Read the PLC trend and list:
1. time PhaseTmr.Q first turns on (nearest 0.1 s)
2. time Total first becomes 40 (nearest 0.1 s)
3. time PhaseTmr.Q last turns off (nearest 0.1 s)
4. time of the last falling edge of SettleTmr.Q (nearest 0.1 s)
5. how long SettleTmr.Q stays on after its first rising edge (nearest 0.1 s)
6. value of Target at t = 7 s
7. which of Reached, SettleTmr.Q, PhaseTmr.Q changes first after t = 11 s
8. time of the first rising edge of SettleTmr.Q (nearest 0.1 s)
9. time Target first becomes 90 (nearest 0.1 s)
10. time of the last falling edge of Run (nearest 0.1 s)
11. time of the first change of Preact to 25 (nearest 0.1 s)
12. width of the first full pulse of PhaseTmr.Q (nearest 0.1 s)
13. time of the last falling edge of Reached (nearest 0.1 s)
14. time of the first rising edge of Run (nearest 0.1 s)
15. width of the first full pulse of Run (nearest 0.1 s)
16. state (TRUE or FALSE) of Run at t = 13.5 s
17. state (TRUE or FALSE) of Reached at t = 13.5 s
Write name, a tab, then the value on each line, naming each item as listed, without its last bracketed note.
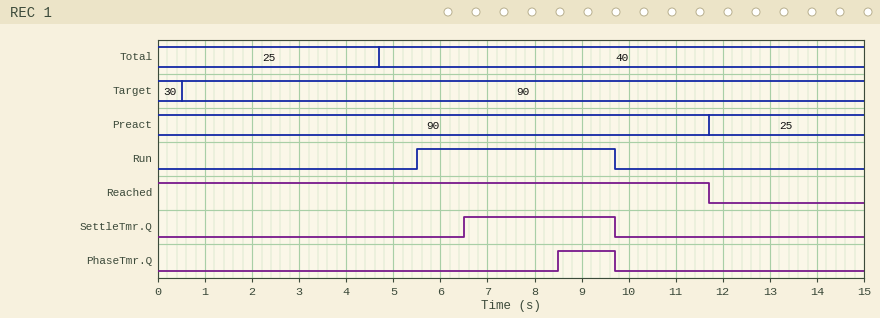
time PhaseTmr.Q first turns on	8.5 s
time Total first becomes 40	4.7 s
time PhaseTmr.Q last turns off	9.7 s
time of the last falling edge of SettleTmr.Q	9.7 s
how long SettleTmr.Q stays on after its first rising edge	3.2 s
value of Target at t = 7 s	90
which of Reached, SettleTmr.Q, PhaseTmr.Q changes first after t = 11 s	Reached
time of the first rising edge of SettleTmr.Q	6.5 s
time Target first becomes 90	0.5 s
time of the last falling edge of Run	9.7 s
time of the first change of Preact to 25	11.7 s
width of the first full pulse of PhaseTmr.Q	1.2 s
time of the last falling edge of Reached	11.7 s
time of the first rising edge of Run	5.5 s
width of the first full pulse of Run	4.2 s
state (TRUE or FALSE) of Run at t = 13.5 s	FALSE
state (TRUE or FALSE) of Reached at t = 13.5 s	FALSE
